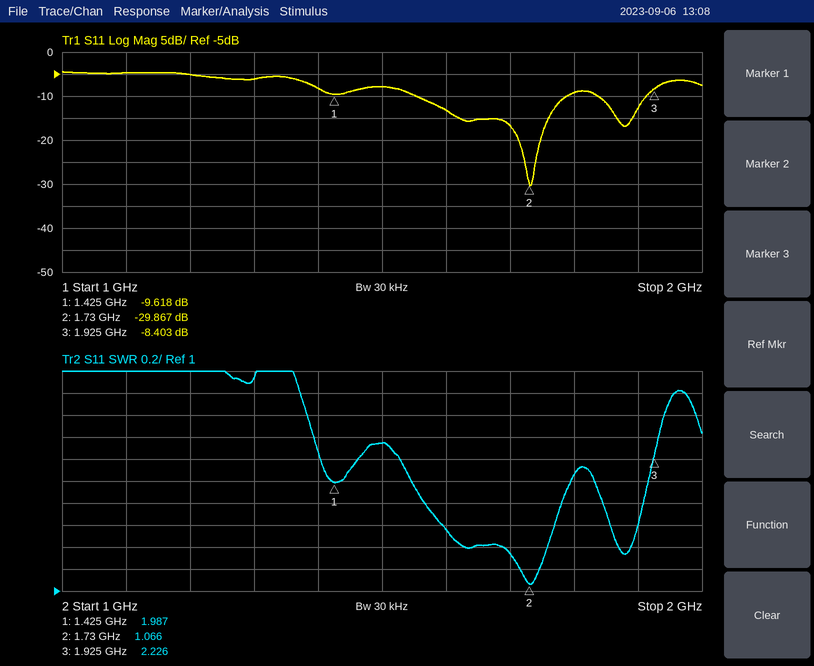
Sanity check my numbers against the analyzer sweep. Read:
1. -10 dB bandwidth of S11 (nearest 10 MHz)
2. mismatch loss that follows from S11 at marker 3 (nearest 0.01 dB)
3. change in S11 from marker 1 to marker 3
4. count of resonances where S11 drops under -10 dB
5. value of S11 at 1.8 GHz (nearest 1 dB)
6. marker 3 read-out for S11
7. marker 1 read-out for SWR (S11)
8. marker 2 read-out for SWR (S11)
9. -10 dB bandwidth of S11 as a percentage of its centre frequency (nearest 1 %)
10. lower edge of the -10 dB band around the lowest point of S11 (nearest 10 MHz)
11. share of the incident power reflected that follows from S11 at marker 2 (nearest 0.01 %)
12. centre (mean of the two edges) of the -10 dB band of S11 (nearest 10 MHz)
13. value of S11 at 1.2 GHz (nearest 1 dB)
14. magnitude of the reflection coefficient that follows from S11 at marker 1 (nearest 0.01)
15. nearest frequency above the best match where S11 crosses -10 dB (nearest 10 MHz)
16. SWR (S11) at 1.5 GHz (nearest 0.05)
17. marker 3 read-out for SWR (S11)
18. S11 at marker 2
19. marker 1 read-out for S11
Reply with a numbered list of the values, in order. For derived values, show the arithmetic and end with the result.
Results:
1. 1.79 GHz − 1.55 GHz = 240 MHz
2. −10 log10(1 − 10^(-8.403/10)) ≈ 0.68 dB
3. -8.403 − (-9.618) = 1.215 dB
4. 2
5. -9 dB
6. -8.403 dB
7. 1.987
8. 1.066
9. 240 MHz / 1.67 GHz ≈ 14 %
10. 1.55 GHz
11. 10^(-29.867/10) ≈ 0.10 %
12. 1.67 GHz
13. -5 dB
14. 10^(-9.618/20) ≈ 0.33
15. 1.79 GHz
16. 2.35
17. 2.226
18. -29.867 dB
19. -9.618 dB
